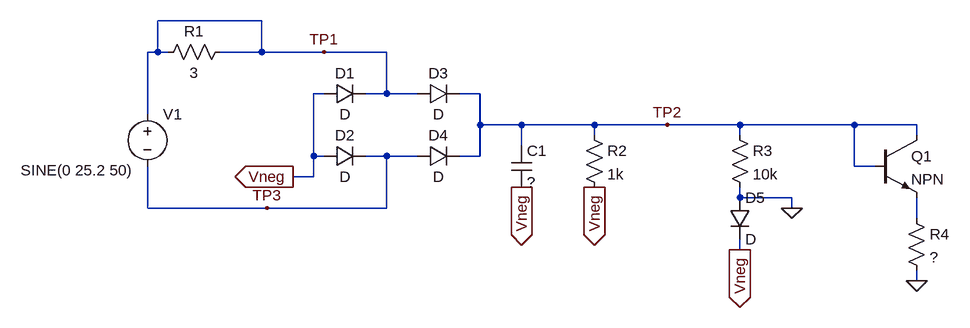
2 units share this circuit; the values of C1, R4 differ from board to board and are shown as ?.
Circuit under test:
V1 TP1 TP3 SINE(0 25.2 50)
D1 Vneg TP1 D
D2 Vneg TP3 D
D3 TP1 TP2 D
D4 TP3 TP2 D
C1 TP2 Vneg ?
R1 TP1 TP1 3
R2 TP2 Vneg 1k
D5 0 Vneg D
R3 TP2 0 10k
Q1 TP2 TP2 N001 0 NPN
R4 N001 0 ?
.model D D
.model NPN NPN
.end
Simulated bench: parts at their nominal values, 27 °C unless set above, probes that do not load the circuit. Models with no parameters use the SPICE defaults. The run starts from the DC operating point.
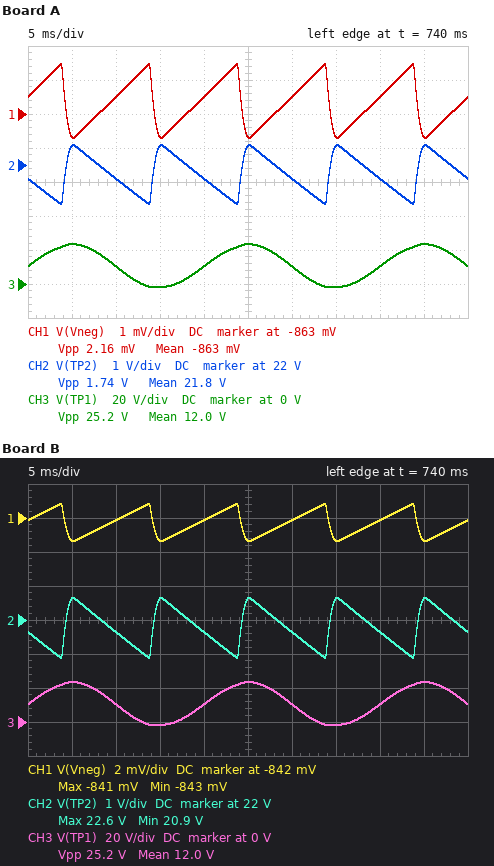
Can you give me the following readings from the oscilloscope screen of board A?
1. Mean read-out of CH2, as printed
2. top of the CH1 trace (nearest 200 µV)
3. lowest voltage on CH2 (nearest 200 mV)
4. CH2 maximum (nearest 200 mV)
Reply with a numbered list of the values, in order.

1. 21.8 V
2. -861.6 mV
3. 20.8 V
4. 22.6 V
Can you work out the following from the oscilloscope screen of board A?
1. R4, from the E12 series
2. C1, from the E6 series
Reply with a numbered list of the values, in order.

1. 6.8 Ω
2. 15 mF
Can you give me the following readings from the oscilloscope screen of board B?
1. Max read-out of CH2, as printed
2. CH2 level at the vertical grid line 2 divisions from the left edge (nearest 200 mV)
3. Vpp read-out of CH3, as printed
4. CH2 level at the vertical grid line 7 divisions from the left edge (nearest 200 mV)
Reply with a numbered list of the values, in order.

1. 22.6 V
2. 21.6 V
3. 25.2 V
4. 22.6 V
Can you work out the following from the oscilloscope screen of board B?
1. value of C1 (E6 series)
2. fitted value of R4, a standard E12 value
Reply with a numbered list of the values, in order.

1. 6.8 mF
2. 15 Ω
